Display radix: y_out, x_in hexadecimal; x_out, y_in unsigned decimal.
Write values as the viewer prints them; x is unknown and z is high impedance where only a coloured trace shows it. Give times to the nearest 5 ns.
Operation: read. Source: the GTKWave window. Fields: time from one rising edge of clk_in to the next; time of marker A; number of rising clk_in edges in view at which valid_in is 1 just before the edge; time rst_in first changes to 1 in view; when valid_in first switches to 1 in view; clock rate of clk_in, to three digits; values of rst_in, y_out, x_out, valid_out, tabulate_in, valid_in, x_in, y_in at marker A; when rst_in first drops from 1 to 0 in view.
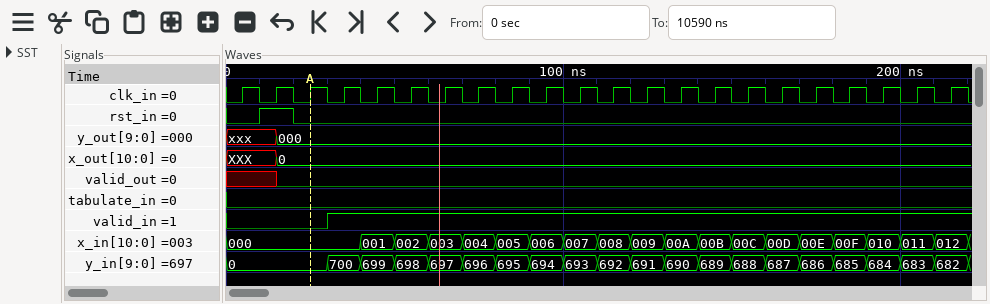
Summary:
10 ns
25 ns
19
10 ns
30 ns
100 MHz
rst_in=0, y_out=000, x_out=0, valid_out=0, tabulate_in=0, valid_in=0, x_in=000, y_in=0
20 ns
